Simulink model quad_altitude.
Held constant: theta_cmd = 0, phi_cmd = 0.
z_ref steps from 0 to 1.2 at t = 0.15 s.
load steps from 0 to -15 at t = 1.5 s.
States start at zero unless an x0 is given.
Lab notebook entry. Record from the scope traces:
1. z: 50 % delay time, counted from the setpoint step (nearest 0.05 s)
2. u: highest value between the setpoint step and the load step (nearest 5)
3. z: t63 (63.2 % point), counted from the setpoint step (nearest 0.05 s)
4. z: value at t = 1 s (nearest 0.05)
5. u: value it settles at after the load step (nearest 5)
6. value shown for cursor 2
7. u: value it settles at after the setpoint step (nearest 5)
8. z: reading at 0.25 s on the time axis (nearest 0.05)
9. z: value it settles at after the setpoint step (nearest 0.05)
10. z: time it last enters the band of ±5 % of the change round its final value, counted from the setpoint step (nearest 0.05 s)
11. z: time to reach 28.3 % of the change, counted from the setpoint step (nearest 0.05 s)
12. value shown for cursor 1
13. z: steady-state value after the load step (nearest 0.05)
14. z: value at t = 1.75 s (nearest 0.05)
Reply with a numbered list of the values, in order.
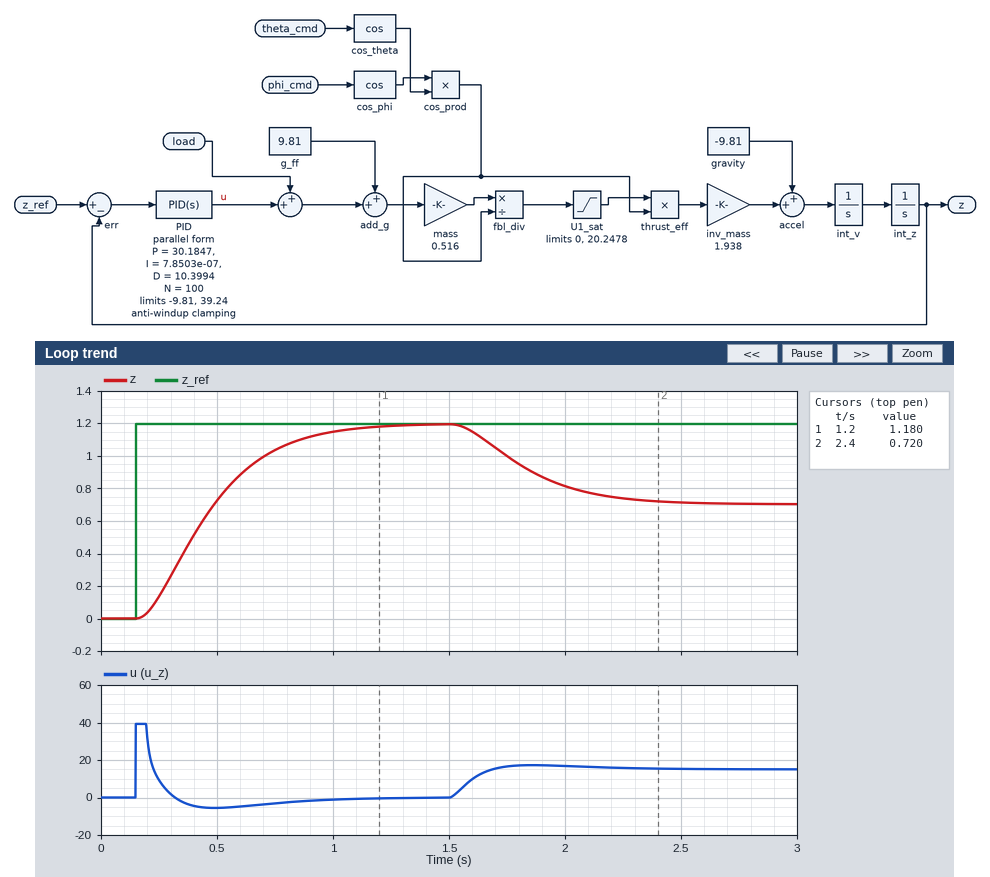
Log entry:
1. 0.30 s
2. 40
3. 0.35 s
4. 1.15
5. 15
6. 0.720
7. 0
8. 0.15
9. 1.20
10. 0.80 s
11. 0.20 s
12. 1.180
13. 0.70
14. 1.00
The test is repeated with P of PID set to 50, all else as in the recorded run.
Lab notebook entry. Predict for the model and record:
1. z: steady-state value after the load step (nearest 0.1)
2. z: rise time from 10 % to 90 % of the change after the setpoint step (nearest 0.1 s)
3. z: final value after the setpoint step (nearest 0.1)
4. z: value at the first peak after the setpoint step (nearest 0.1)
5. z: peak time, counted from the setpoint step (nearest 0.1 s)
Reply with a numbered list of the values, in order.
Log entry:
1. 0.9
2. 0.3 s
3. 1.2
4. 1.3
5. 0.6 s
